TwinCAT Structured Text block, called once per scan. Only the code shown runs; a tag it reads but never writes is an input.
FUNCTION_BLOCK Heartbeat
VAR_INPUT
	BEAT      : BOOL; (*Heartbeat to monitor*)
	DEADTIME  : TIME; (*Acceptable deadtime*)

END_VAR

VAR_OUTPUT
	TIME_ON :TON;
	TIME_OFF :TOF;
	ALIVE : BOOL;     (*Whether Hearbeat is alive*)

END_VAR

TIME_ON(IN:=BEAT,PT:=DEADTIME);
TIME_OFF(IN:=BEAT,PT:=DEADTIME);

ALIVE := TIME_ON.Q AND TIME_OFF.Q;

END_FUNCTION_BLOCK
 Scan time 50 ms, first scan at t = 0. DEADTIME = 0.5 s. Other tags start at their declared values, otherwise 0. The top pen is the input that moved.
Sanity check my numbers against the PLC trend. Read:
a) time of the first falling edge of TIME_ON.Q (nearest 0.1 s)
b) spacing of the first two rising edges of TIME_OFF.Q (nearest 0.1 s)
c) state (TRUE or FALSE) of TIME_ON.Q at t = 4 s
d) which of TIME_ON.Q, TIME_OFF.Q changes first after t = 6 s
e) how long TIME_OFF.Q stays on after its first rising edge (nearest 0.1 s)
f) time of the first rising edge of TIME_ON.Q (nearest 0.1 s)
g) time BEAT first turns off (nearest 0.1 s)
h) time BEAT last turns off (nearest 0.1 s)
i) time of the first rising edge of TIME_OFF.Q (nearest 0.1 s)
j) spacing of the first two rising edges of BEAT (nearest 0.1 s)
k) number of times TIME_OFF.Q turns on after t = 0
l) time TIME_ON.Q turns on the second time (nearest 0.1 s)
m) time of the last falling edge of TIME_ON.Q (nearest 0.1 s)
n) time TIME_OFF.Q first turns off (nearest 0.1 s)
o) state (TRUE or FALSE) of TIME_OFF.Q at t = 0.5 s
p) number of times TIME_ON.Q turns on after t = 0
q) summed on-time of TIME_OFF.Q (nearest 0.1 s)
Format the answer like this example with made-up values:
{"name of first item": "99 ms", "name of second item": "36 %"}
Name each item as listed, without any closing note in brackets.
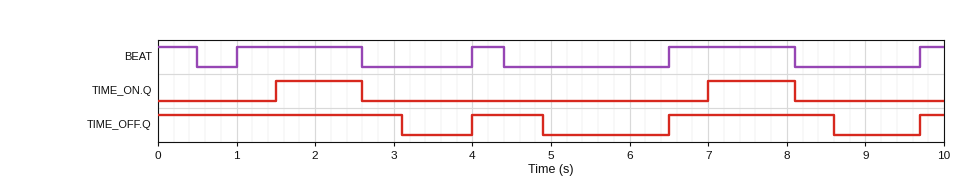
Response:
{"time of the first falling edge of TIME_ON.Q": "2.6 s", "spacing of the first two rising edges of TIME_OFF.Q": "2.5 s", "state (TRUE or FALSE) of TIME_ON.Q at t = 4 s": "FALSE", "which of TIME_ON.Q, TIME_OFF.Q changes first after t = 6 s": "TIME_OFF.Q", "how long TIME_OFF.Q stays on after its first rising edge": "0.9 s", "time of the first rising edge of TIME_ON.Q": "1.5 s", "time BEAT first turns off": "0.5 s", "time BEAT last turns off": "8.1 s", "time of the first rising edge of TIME_OFF.Q": "4.0 s", "spacing of the first two rising edges of BEAT": "3.0 s", "number of times TIME_OFF.Q turns on after t = 0": "3", "time TIME_ON.Q turns on the second time": "7.0 s", "time of the last falling edge of TIME_ON.Q": "8.1 s", "time TIME_OFF.Q first turns off": "3.1 s", "state (TRUE or FALSE) of TIME_OFF.Q at t = 0.5 s": "TRUE", "number of times TIME_ON.Q turns on after t = 0": "2", "summed on-time of TIME_OFF.Q": "6.4 s"}
